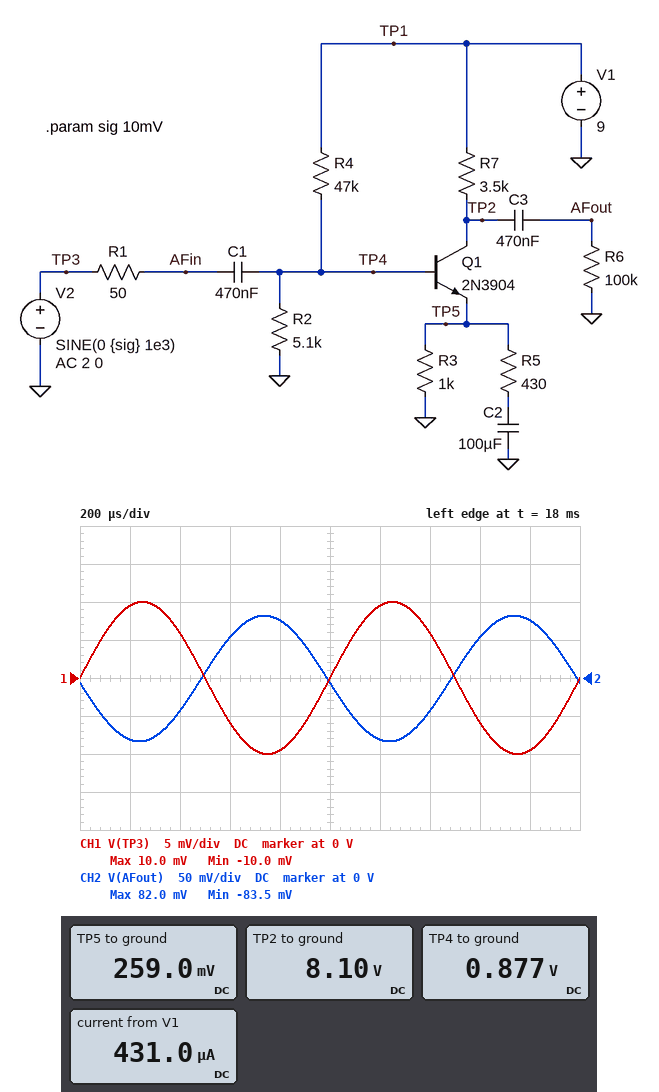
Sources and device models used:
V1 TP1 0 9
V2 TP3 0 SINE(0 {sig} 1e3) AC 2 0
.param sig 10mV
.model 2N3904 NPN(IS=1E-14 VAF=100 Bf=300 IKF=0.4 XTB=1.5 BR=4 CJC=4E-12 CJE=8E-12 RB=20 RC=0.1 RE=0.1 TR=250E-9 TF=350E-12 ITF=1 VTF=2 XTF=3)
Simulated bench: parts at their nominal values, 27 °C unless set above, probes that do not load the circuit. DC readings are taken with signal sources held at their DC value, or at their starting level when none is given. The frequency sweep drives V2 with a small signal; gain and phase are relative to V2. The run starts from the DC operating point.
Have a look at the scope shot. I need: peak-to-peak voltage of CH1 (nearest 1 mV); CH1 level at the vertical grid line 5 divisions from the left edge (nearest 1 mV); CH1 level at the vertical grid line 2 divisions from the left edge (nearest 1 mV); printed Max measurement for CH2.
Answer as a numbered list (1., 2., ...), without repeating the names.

1. 20 mV
2. 0 V
3. 6 mV
4. 82.0 mV
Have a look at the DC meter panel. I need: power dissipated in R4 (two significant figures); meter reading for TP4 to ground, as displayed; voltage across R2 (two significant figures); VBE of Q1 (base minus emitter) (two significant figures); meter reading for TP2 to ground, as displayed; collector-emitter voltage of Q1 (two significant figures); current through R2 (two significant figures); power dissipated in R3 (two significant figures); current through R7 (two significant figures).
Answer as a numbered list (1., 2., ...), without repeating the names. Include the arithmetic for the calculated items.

1. (9 V - 877 mV)^2 / 47 kΩ = 1.4 mW
2. 0.877 V
3. 877 mV = 880 mV
4. 877 mV - 259 mV = 620 mV
5. 8.10 V
6. 8.1 V - 259 mV = 7.8 V
7. (877 mV) / 5.1 kΩ = 170 µA
8. (259 mV)^2 / 1 kΩ = 67 µW
9. (9 V - 8.1 V) / 3.5 kΩ = 260 µA
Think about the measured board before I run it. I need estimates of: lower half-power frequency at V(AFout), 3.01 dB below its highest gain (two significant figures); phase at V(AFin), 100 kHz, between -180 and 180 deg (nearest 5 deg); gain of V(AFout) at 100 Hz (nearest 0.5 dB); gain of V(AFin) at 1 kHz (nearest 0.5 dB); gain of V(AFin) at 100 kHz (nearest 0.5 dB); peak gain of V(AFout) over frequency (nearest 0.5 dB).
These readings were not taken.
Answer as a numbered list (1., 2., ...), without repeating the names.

1. 76 Hz
2. 0 deg
3. 16.5 dB
4. 0 dB
5. 0 dB
6. 18.5 dB
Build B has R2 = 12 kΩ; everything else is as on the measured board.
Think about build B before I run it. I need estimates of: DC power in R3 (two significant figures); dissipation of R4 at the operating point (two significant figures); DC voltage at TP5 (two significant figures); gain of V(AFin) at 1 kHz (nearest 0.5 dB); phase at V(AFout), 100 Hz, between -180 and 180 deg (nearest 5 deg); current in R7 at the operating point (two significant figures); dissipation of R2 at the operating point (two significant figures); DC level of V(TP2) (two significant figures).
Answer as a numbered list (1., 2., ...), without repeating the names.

1. 1.3 mW
2. 1.1 mW
3. 1.1 V
4. 0 dB
5. -155 deg
6. 1.1 mA
7. 270 µW
8. 5.0 V
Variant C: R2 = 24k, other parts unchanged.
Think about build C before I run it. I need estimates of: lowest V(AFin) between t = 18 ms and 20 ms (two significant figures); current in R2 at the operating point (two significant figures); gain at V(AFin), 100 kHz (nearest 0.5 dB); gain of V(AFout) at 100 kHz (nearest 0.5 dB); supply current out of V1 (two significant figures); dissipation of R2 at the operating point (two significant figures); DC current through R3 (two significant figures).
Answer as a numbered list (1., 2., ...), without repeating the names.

1. -9.4 mV
2. 110 µA
3. -1.0 dB
4. 5.5 dB
5. 2.1 mA
6. 300 µW
7. 2.0 mA
